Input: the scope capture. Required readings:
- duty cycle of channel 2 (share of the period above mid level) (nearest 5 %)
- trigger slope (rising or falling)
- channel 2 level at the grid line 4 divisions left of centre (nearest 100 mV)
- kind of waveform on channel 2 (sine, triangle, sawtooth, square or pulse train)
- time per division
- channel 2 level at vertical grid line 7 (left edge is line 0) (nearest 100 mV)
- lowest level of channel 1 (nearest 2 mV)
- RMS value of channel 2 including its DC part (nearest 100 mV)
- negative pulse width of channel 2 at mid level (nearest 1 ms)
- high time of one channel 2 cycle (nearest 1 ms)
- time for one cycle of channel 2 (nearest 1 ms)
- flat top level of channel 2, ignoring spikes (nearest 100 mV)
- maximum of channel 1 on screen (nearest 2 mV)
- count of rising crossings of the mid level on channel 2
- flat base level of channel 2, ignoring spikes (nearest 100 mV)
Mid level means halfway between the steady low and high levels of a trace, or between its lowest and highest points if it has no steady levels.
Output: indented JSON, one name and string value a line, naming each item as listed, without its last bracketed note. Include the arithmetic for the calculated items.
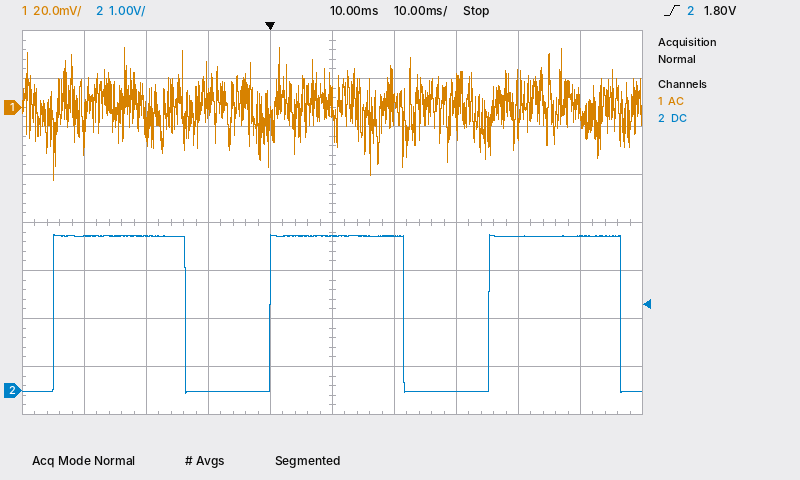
{
  "duty cycle of channel 2 (share of the period above mid level)": "21 ms / 35 ms ≈ 60 %",
  "trigger slope": "rising",
  "channel 2 level at the grid line 4 divisions left of centre": "3.2 V",
  "kind of waveform on channel 2": "pulse train",
  "time per division": "10 ms",
  "channel 2 level at vertical grid line 7 (left edge is line 0)": "0.0 V",
  "lowest level of channel 1": "-30 mV",
  "RMS value of channel 2 including its DC part": "√(0.6 × (3.2 V)² + 0.4 × (0.0 V)²) ≈ 2.5 V",
  "negative pulse width of channel 2 at mid level": "14 ms",
  "high time of one channel 2 cycle": "21 ms",
  "time for one cycle of channel 2": "35 ms",
  "flat top level of channel 2, ignoring spikes": "3.2 V",
  "maximum of channel 1 on screen": "24 mV",
  "count of rising crossings of the mid level on channel 2": "3",
  "flat base level of channel 2, ignoring spikes": "0.0 V"
}
